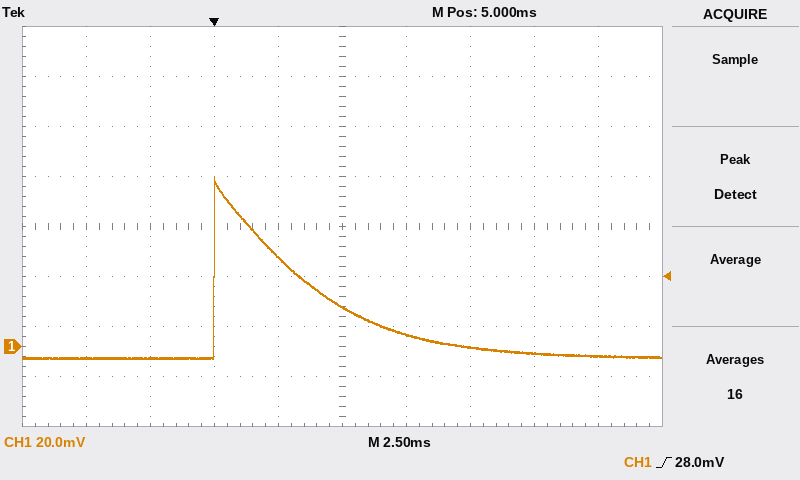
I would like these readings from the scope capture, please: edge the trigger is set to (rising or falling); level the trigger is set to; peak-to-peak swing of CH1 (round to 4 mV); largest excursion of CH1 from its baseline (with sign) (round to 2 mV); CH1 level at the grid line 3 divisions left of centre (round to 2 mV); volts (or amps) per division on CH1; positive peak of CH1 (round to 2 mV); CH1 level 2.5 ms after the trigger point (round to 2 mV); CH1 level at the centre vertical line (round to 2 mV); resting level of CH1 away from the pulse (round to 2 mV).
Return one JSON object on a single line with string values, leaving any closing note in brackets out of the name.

{"edge the trigger is set to": "rising", "level the trigger is set to": "28.0 mV", "peak-to-peak swing of CH1": "72 mV", "largest excursion of CH1 from its baseline (with sign)": "+72 mV", "CH1 level at the grid line 3 divisions left of centre": "-4 mV", "volts (or amps) per division on CH1": "20 mV", "positive peak of CH1": "68 mV", "CH1 level 2.5 ms after the trigger point": "36 mV", "CH1 level at the centre vertical line": "16 mV", "resting level of CH1 away from the pulse": "-4 mV"}
